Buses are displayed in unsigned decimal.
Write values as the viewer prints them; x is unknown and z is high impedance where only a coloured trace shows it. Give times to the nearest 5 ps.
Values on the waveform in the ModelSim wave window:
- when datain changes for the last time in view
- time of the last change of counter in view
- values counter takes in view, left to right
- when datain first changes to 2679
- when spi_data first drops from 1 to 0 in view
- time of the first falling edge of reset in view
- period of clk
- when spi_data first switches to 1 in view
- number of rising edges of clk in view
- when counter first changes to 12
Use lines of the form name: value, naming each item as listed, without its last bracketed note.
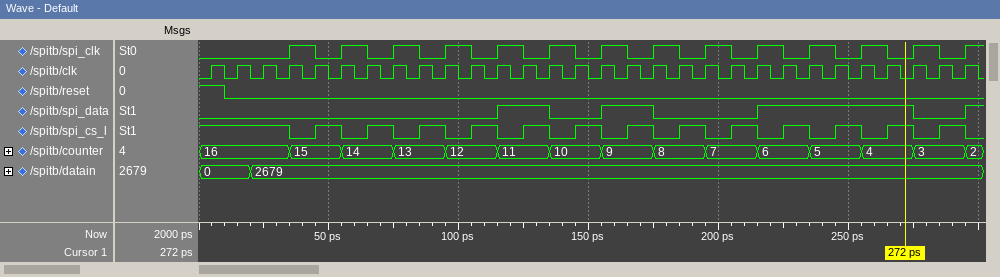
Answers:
when datain changes for the last time in view: 20 ps
time of the last change of counter in view: 295 ps
values counter takes in view, left to right: 16, 15, 14, 13, 12, 11, 10, 9, 8, 7, 6, 5, 4, 3, 2
when datain first changes to 2679: 20 ps
when spi_data first drops from 1 to 0 in view: 135 ps
time of the first falling edge of reset in view: 10 ps
period of clk: 10 ps
when spi_data first switches to 1 in view: 115 ps
number of rising edges of clk in view: 30
when counter first changes to 12: 95 ps
